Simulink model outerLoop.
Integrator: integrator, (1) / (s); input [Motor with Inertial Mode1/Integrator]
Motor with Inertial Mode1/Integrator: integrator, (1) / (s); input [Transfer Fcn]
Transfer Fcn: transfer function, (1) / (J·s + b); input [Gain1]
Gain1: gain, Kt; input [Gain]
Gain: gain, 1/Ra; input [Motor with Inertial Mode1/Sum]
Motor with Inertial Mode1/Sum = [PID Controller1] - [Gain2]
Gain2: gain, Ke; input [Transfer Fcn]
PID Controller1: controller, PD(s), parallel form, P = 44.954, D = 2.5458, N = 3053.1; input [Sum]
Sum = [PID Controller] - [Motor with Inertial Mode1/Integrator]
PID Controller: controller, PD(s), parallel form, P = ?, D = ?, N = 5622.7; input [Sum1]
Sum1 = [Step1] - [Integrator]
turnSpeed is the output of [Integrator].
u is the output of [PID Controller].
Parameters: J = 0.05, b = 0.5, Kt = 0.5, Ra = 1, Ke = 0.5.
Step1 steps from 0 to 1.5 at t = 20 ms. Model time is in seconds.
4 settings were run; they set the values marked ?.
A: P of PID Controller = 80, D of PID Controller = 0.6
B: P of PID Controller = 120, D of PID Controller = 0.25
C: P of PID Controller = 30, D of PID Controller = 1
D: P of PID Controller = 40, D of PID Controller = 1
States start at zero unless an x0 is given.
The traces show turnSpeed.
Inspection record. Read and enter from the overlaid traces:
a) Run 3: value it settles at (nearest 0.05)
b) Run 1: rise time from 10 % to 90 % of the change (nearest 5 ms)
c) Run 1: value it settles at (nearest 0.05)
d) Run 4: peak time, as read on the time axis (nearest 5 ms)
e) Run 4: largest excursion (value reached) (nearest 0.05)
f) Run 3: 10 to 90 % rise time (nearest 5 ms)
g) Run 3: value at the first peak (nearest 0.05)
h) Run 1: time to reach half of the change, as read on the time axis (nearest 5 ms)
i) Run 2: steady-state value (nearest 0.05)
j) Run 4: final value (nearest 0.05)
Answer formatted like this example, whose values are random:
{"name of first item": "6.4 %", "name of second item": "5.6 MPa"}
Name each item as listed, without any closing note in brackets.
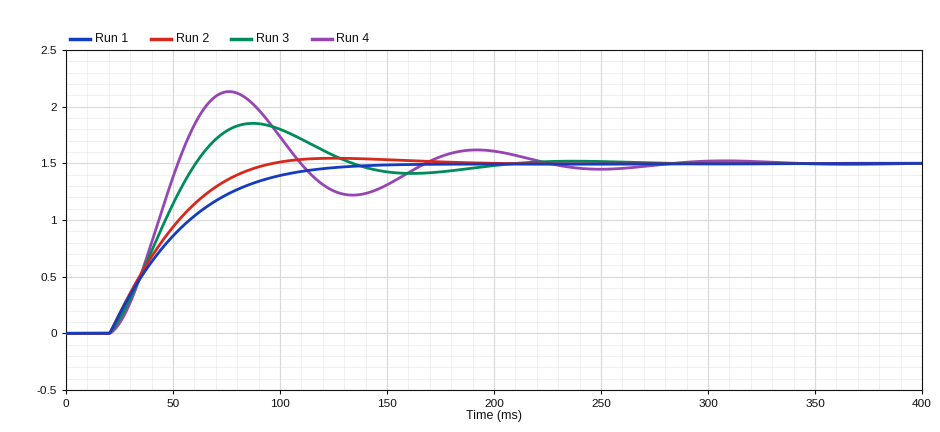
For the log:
{"Run 3: value it settles at": "1.50", "Run 1: rise time from 10 % to 90 % of the change": "65 ms", "Run 1: value it settles at": "1.50", "Run 4: peak time, as read on the time axis": "75 ms", "Run 4: largest excursion (value reached)": "2.15", "Run 3: 10 to 90 % rise time": "30 ms", "Run 3: value at the first peak": "1.85", "Run 1: time to reach half of the change, as read on the time axis": "45 ms", "Run 2: steady-state value": "1.50", "Run 4: final value": "1.50"}
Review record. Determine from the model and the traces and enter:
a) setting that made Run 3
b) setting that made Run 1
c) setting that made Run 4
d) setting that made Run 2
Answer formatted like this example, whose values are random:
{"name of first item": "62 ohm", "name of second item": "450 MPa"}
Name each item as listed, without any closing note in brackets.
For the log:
{"setting that made Run 3": "A", "setting that made Run 1": "C", "setting that made Run 4": "B", "setting that made Run 2": "D"}
